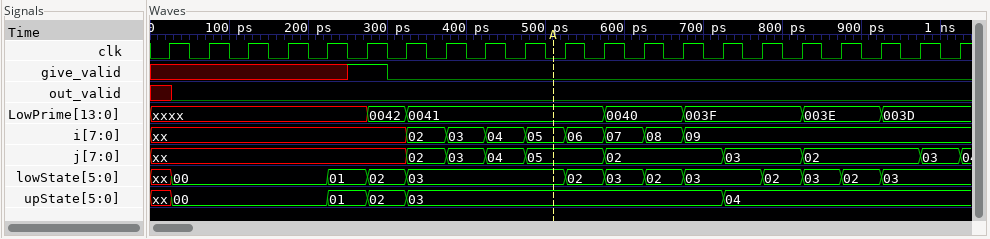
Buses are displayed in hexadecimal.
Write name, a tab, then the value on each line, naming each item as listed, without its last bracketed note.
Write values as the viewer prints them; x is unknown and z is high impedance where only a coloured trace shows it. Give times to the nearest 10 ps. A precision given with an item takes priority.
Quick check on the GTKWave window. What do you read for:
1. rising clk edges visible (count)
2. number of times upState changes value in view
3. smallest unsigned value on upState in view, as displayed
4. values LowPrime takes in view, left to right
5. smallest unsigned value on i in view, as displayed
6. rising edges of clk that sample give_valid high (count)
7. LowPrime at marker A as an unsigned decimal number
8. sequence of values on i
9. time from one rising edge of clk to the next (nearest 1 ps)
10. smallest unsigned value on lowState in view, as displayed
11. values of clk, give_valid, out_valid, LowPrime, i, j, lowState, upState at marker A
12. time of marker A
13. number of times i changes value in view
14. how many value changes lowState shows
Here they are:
rising clk edges visible	21
number of times upState changes value in view	5
smallest unsigned value on upState in view, as displayed	00
values LowPrime takes in view, left to right	xxxx, 0042, 0041, 0040, 003F, 003E, 003D
smallest unsigned value on i in view, as displayed	02
rising edges of clk that sample give_valid high	1
LowPrime at marker A as an unsigned decimal number	65
sequence of values on i	xx, 02, 03, 04, 05, 06, 07, 08, 09
time from one rising edge of clk to the next	50 ps
smallest unsigned value on lowState in view, as displayed	00
values of clk, give_valid, out_valid, LowPrime, i, j, lowState, upState at marker A	clk=0, give_valid=0, out_valid=0, LowPrime=0041, i=05, j=05, lowState=03, upState=03
time of marker A	510 ps
number of times i changes value in view	8
how many value changes lowState shows	12
